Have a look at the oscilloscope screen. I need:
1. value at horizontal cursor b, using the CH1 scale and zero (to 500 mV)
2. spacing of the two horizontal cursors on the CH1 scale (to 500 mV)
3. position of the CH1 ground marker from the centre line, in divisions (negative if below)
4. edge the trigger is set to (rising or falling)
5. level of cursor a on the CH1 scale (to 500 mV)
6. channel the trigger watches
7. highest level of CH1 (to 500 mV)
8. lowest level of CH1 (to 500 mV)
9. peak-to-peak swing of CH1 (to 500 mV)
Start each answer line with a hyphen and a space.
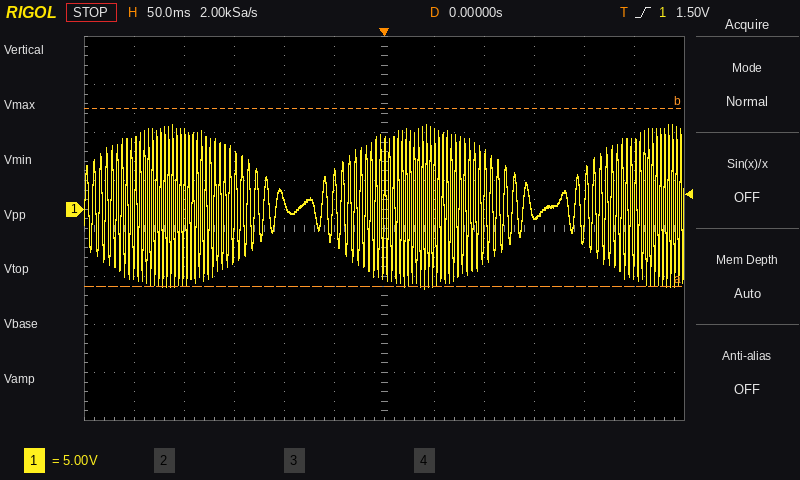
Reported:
- 10.5 V
- 18.5 V
- +0.4 div
- rising
- -8.0 V
- CH1
- 9.0 V
- -8.0 V
- 17.0 V
